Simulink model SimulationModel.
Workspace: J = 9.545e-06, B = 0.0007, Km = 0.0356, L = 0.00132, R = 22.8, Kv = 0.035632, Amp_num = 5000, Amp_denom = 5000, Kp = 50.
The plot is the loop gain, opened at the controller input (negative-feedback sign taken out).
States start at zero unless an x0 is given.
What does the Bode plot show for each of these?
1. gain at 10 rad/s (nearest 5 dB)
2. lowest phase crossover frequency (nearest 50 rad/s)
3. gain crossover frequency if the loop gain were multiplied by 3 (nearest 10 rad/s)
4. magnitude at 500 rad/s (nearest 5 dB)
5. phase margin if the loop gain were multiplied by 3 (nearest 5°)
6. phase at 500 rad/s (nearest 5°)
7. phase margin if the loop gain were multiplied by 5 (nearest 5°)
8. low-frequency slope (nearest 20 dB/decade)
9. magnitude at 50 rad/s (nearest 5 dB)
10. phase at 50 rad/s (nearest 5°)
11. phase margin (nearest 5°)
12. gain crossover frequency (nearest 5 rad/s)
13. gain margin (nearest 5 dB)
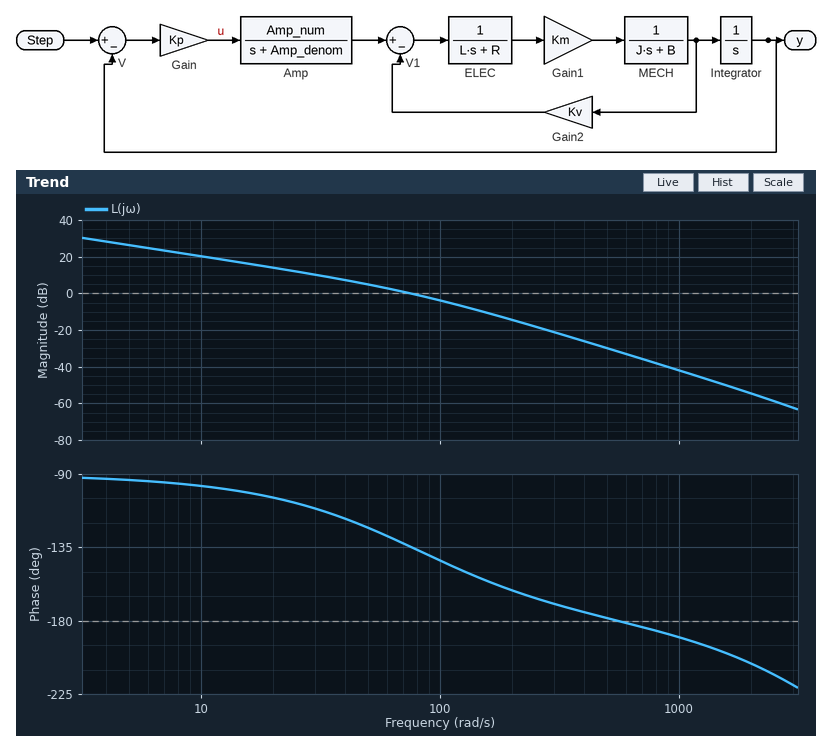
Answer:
20 dB
550 rad/s
150 rad/s
-30 dB
25°
-180°
20°
-20 dB/decade
5 dB
-125°
45°
75 rad/s
30 dB
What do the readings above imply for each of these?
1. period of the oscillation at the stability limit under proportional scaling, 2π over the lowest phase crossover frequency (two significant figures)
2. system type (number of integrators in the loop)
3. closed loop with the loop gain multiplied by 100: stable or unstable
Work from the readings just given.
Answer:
0.011 s
1
unstable
